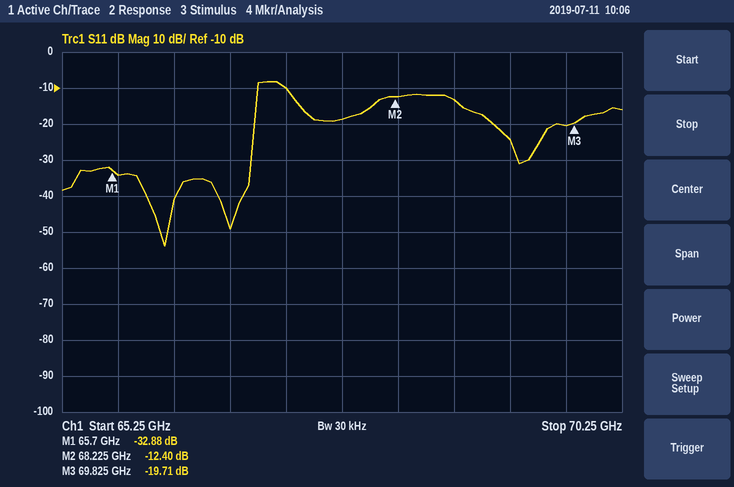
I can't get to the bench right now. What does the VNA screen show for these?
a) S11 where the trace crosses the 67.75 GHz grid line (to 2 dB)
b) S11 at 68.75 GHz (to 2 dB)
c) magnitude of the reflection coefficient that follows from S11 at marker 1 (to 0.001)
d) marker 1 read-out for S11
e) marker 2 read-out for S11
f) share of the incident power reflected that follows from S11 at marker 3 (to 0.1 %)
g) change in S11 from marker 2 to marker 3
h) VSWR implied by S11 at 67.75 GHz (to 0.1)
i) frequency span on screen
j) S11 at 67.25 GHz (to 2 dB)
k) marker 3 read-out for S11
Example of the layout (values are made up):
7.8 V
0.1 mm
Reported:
-18 dB
-14 dB
0.023
-32.88 dB
-12.40 dB
1.1 %
-7.31 dB
1.3
5 GHz
-10 dB
-19.71 dB
